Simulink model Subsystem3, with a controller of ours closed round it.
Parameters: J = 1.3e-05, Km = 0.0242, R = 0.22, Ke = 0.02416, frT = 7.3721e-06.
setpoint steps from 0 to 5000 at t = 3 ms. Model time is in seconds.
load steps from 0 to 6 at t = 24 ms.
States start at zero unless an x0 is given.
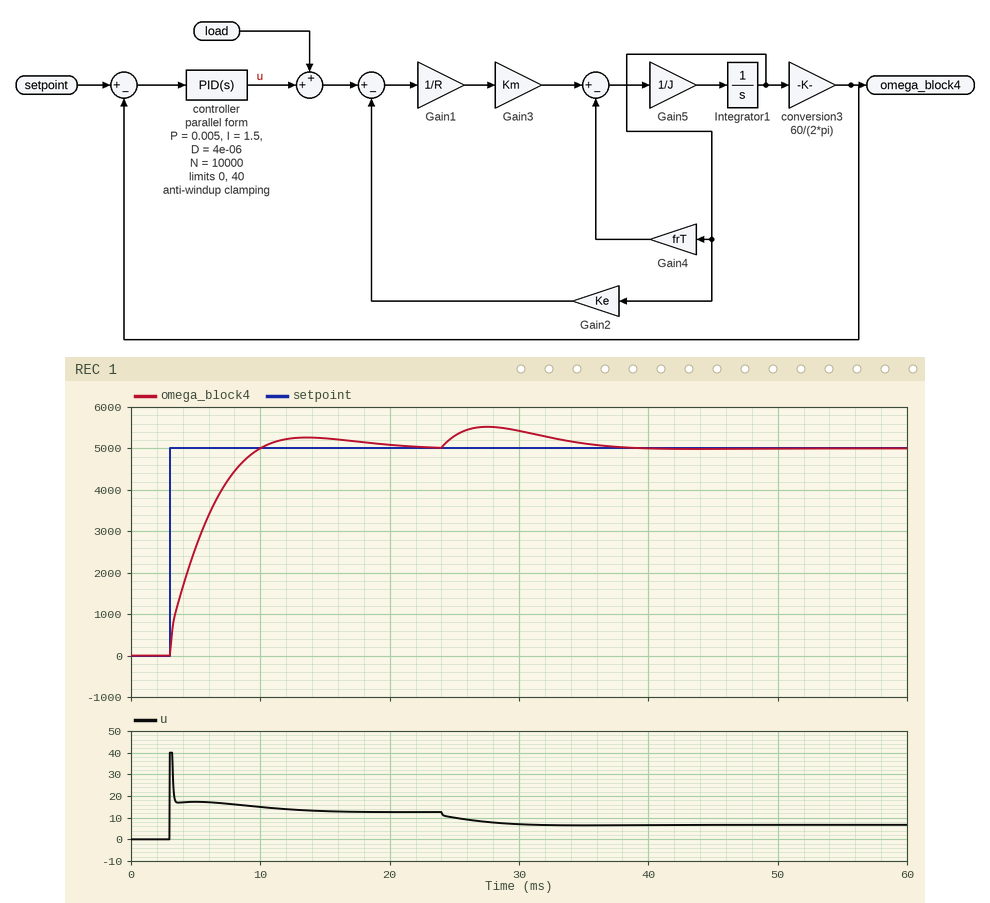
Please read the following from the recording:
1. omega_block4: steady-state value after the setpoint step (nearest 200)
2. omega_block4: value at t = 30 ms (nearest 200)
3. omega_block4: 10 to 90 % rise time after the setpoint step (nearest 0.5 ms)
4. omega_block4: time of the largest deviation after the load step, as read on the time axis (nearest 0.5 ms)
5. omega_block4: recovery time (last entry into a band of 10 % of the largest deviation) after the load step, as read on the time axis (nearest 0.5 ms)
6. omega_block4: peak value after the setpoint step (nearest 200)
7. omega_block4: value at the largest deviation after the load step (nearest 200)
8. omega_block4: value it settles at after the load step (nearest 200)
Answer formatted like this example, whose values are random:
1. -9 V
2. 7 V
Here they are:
1. 5000
2. 5400
3. 5.0 ms
4. 27.5 ms
5. 37.0 ms
6. 5200
7. 5600
8. 5000
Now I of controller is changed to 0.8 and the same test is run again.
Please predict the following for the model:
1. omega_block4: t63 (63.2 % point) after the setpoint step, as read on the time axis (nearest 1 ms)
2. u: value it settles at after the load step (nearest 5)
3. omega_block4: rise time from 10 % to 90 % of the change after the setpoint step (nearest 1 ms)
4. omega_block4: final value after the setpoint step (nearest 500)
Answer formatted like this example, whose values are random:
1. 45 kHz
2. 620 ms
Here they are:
1. 6 ms
2. 5
3. 8 ms
4. 5000
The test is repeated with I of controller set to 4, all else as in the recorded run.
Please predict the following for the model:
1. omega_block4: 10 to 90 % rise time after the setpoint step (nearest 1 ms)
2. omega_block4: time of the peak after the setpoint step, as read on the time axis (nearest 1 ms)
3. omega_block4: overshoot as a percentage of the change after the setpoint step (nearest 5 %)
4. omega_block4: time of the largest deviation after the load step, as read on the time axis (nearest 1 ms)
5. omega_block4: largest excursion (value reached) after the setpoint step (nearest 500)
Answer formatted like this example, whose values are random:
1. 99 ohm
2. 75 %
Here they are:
1. 3 ms
2. 9 ms
3. 20 %
4. 26 ms
5. 6000
